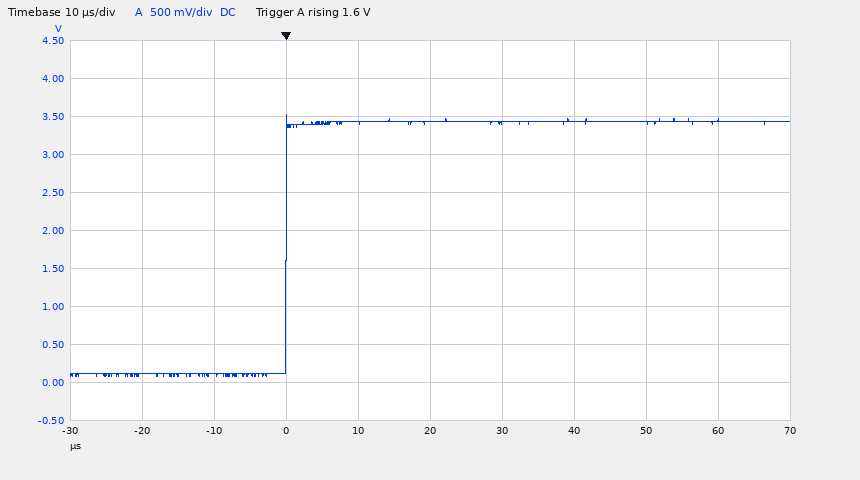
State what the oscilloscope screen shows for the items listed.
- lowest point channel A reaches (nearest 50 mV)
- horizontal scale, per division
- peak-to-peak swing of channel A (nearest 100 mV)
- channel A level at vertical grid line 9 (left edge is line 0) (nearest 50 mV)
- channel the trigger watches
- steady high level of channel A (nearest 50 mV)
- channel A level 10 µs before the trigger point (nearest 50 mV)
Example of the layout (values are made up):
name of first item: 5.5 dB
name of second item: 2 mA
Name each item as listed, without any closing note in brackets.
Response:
lowest point channel A reaches: 100 mV
horizontal scale, per division: 10 µs
peak-to-peak swing of channel A: 3.40 V
channel A level at vertical grid line 9 (left edge is line 0): 3.45 V
channel the trigger watches: channel A
steady high level of channel A: 3.45 V
channel A level 10 µs before the trigger point: 100 mV
